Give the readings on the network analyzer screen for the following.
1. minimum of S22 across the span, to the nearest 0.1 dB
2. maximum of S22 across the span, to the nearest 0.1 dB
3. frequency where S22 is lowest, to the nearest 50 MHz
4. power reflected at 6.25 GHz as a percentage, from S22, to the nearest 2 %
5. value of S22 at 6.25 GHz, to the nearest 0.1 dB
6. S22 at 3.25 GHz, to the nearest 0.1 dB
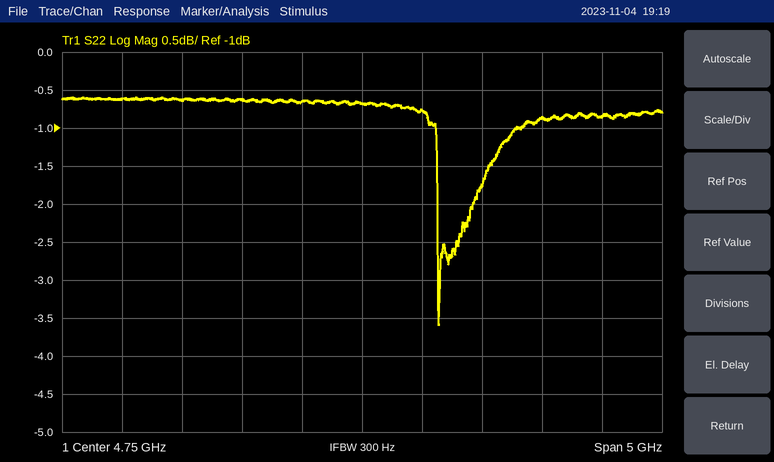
-3.6 dB
-0.6 dB
5.40 GHz
82 %
-0.9 dB
-0.6 dB
